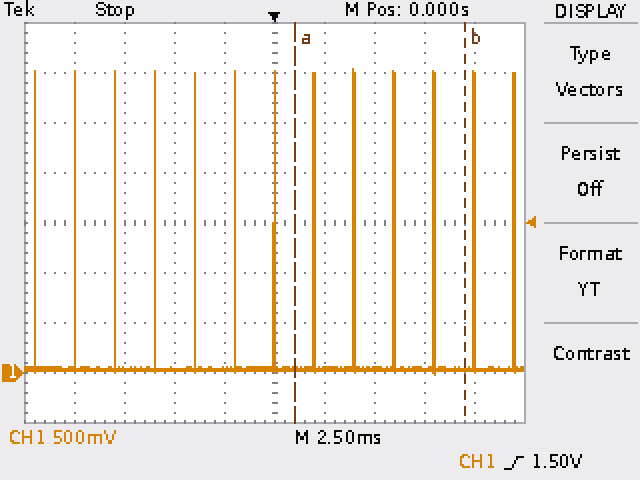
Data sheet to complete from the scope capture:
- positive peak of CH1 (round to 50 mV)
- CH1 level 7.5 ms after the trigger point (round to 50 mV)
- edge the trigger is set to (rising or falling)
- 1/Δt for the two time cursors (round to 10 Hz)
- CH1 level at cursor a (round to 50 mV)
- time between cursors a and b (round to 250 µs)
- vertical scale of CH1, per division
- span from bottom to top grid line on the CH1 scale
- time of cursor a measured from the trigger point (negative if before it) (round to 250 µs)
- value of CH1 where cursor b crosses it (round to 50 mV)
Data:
3.05 V
50 mV
rising
120 Hz
50 mV
8.50 ms
500 mV
4 V
+1.00 ms
50 mV
